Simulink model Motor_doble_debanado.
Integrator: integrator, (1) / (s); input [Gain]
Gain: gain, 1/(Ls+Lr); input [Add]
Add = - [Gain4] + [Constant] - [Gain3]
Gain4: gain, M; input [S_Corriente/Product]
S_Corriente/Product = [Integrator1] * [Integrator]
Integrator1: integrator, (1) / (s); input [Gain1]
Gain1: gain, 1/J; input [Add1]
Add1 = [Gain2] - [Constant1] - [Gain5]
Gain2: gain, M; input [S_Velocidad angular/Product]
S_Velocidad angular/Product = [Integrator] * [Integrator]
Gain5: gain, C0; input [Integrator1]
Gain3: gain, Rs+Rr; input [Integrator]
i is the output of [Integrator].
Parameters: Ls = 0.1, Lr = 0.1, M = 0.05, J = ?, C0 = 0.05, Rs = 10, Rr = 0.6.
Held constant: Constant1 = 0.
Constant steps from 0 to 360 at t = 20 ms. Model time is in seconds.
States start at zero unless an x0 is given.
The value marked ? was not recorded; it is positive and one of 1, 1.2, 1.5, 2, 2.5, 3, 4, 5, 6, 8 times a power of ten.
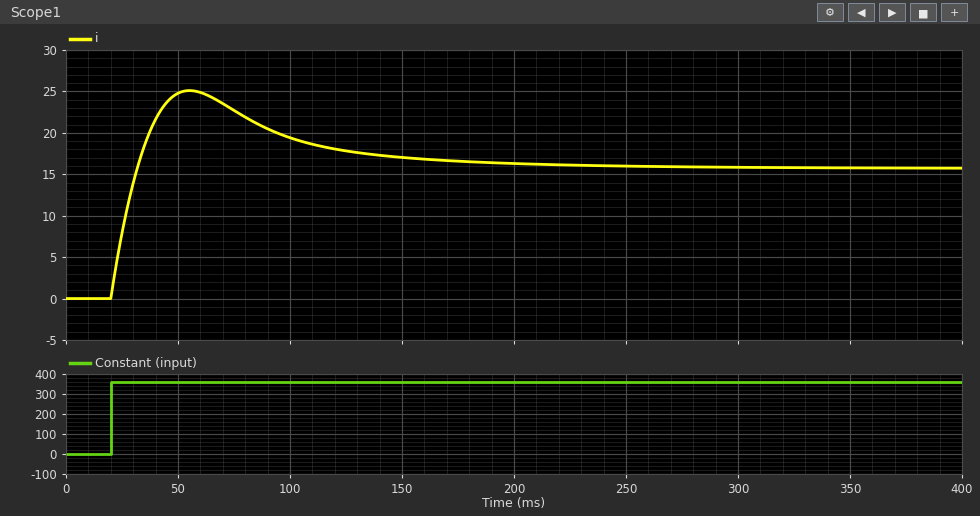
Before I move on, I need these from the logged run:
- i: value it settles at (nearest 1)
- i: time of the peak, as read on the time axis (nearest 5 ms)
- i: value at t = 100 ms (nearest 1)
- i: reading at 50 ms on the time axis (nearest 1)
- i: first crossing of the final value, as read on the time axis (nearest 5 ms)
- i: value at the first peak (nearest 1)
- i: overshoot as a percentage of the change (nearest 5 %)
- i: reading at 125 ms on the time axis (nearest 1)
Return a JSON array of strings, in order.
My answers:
["16", "55 ms", "19", "25", "30 ms", "25", "60 %", "18"]
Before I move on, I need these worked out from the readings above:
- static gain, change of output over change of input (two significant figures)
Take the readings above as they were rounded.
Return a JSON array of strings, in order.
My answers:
["0.044"]
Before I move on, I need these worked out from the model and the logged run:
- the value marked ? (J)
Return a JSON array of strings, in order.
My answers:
["0.008"]
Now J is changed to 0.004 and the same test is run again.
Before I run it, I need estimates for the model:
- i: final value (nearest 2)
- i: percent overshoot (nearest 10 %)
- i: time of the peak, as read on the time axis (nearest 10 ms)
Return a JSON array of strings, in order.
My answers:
["16", "50 %", "50 ms"]
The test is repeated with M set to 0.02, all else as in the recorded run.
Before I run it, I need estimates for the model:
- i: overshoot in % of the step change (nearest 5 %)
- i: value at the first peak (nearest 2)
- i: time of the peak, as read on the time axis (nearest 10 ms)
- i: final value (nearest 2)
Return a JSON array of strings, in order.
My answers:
["25 %", "30", "80 ms", "24"]
